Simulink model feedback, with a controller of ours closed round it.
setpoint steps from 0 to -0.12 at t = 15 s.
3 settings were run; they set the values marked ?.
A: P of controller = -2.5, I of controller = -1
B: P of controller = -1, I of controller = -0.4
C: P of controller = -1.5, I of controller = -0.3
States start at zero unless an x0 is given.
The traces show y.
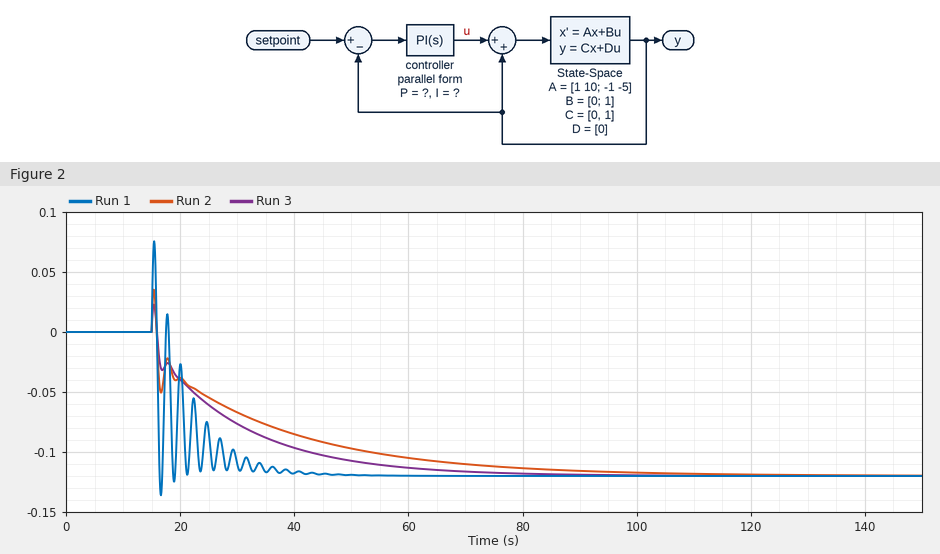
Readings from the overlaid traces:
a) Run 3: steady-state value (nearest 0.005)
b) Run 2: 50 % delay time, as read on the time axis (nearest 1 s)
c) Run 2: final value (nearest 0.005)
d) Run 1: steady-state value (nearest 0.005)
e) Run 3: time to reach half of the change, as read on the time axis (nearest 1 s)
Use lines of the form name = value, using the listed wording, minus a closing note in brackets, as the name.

Run 3: steady-state value = -0.120
Run 2: 50 % delay time, as read on the time axis = 27 s
Run 2: final value = -0.120
Run 1: steady-state value = -0.120
Run 3: time to reach half of the change, as read on the time axis = 25 s
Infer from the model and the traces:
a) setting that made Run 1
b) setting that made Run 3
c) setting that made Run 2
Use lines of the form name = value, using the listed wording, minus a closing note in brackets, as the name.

setting that made Run 1 = A
setting that made Run 3 = B
setting that made Run 2 = C
